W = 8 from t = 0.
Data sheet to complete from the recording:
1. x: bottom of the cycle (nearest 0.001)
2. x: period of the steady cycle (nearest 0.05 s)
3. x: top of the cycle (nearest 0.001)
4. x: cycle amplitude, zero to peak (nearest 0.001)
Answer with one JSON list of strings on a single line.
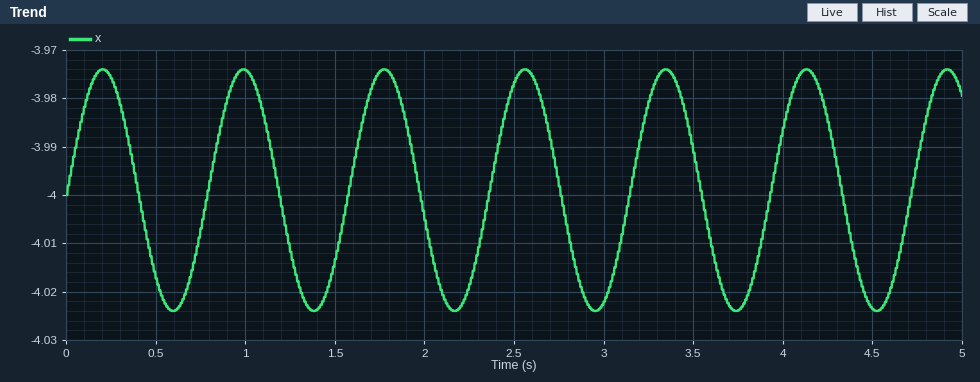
["-4.024", "0.80 s", "-3.974", "0.025"]
